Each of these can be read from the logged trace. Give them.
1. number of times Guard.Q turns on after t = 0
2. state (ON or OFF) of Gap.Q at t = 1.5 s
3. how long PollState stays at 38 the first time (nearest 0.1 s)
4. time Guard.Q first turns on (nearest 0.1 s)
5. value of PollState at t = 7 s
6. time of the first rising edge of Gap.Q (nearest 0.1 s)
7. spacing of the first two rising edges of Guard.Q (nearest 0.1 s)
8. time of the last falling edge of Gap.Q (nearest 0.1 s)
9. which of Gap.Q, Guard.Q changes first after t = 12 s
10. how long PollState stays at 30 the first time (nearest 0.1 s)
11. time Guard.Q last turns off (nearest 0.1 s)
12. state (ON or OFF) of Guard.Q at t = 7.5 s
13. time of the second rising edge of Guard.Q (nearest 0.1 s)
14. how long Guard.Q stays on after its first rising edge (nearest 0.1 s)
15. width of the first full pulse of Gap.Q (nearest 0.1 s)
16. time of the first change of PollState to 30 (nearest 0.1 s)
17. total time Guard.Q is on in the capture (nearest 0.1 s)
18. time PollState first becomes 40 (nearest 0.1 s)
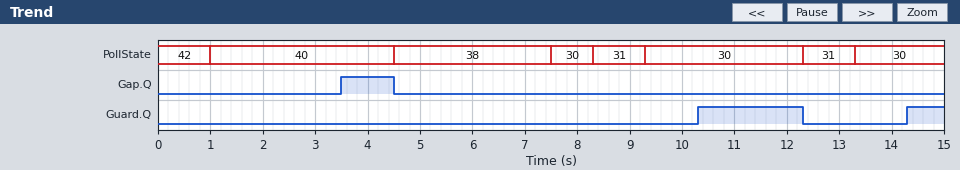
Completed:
2
OFF
3.0 s
10.3 s
38
3.5 s
4.0 s
4.5 s
Guard.Q
0.8 s
12.3 s
OFF
14.3 s
2.0 s
1.0 s
7.5 s
2.7 s
1.0 s
